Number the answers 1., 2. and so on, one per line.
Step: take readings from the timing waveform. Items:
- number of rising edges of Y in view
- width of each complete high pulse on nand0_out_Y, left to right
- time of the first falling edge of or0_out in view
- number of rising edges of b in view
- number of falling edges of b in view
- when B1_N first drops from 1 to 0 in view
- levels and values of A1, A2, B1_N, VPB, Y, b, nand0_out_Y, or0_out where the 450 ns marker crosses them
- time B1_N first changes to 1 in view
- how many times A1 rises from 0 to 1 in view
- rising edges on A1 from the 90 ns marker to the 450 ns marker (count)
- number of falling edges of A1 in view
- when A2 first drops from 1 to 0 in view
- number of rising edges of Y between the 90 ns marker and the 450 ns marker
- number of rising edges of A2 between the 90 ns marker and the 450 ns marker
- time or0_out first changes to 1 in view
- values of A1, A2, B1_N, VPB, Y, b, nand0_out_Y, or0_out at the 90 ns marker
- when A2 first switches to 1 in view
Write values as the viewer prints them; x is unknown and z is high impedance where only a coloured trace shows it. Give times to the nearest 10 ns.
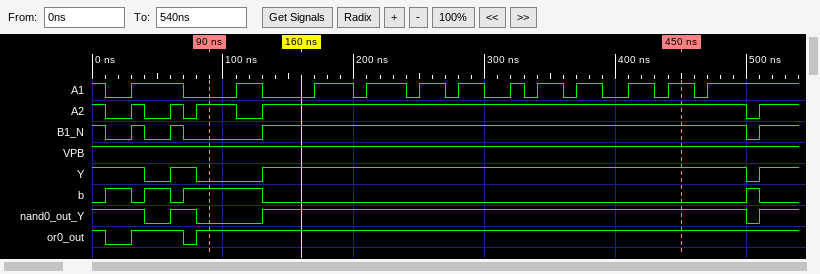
1. 3
2. 20 ns, 370 ns
3. 10 ns
4. 4
5. 4
6. 10 ns
7. A1=1, A2=1, B1_N=1, VPB=1, Y=1, b=0, nand0_out_Y=1, or0_out=1
8. 30 ns
9. 12
10. 10
11. 12
12. 10 ns
13. 1
14. 1
15. 30 ns
16. A1=0, A2=1, B1_N=0, VPB=1, Y=0, b=1, nand0_out_Y=0, or0_out=1
17. 30 ns
